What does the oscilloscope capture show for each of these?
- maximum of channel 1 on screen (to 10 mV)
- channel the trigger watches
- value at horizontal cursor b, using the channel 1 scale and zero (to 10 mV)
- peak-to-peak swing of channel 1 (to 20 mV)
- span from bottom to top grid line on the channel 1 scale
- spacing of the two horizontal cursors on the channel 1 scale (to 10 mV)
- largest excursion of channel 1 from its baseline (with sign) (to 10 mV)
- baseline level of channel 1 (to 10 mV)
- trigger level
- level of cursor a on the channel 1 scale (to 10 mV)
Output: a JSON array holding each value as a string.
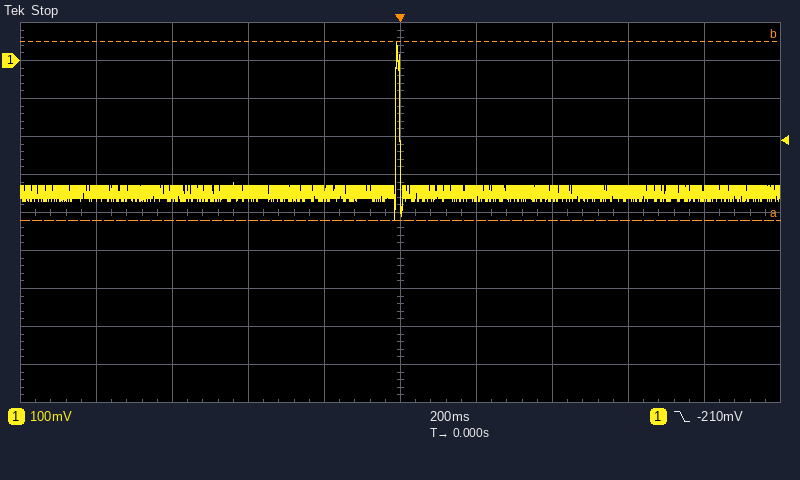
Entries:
["50 mV", "channel 1", "50 mV", "460 mV", "1 V", "470 mV", "+390 mV", "-340 mV", "-210 mV", "-420 mV"]
